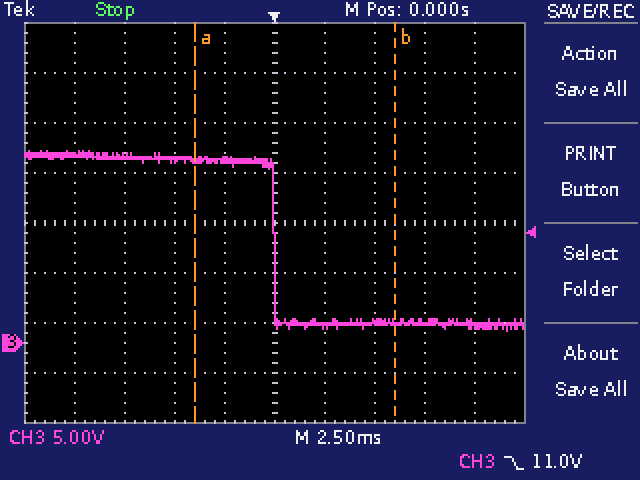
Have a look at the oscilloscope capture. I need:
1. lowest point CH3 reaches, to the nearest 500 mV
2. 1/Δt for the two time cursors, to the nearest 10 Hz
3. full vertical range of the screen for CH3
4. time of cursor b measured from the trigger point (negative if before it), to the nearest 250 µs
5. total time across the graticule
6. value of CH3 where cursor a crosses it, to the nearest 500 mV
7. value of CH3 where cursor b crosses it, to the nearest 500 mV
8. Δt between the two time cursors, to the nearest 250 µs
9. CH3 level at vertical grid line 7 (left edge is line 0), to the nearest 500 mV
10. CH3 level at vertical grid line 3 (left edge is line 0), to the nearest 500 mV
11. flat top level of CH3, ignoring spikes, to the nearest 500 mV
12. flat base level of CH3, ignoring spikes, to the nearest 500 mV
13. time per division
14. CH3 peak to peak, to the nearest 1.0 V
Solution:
1.0 V
100 Hz
40 V
+6.00 ms
25 ms
18.5 V
2.0 V
10.00 ms
2.0 V
18.5 V
18.5 V
2.0 V
2.5 ms
18.0 V
